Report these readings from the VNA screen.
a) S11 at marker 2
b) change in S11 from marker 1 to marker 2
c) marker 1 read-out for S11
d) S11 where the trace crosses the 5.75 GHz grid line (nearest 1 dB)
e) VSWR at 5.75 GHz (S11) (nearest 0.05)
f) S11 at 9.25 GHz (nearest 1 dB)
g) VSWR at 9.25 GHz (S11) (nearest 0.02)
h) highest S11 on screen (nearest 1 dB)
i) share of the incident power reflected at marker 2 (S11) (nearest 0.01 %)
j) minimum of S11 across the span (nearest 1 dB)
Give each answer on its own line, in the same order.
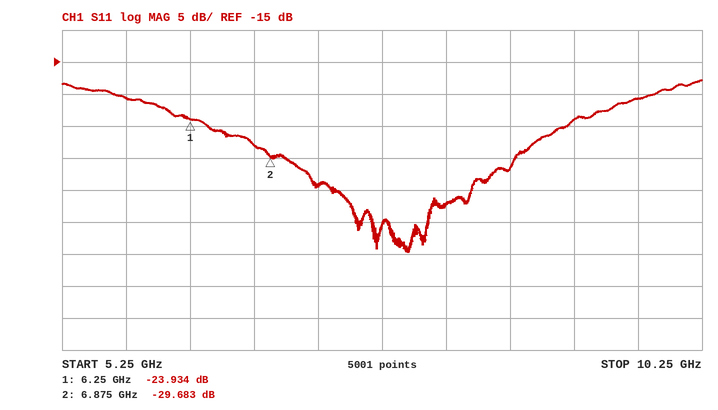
-29.683 dB
-5.749 dB
-23.934 dB
-21 dB
1.20
-24 dB
1.14
-18 dB
0.11 %
-45 dB
